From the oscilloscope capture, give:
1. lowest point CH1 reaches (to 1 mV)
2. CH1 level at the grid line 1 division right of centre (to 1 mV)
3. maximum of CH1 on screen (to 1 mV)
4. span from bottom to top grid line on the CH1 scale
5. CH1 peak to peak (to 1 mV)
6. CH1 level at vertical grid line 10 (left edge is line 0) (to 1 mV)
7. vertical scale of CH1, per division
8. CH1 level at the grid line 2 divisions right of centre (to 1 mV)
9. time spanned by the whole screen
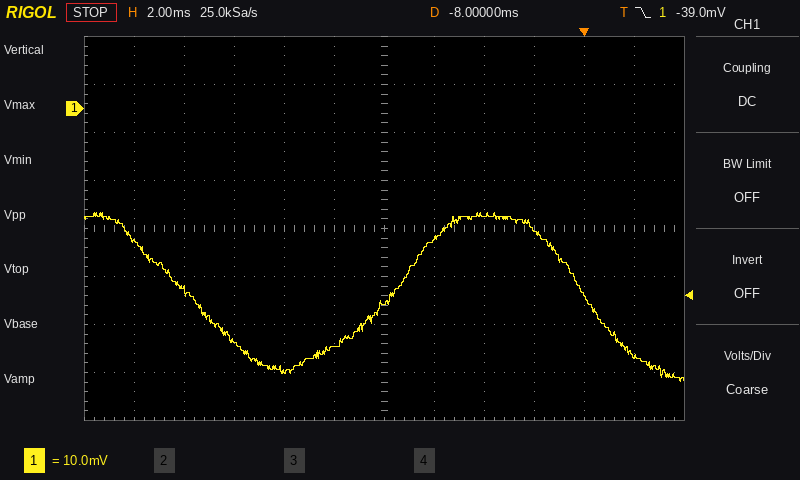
-57 mV
-27 mV
-22 mV
80 mV
35 mV
-39 mV
10 mV
-22 mV
24 ms
